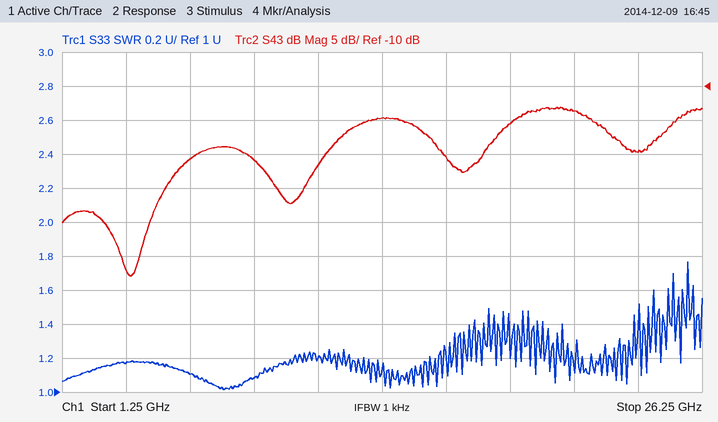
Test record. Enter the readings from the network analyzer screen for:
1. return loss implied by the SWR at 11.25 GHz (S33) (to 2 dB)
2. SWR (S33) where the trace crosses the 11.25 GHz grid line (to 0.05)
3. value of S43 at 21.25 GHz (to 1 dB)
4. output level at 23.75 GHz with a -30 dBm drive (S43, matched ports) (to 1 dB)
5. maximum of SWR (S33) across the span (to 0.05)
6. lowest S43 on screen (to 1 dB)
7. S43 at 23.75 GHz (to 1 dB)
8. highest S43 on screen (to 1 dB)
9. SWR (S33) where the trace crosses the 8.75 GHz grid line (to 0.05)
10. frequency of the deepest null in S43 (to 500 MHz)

20 dB
1.20
-14 dB
-50 dBm
1.75
-38 dB
-20 dB
-13 dB
1.10
4.0 GHz
